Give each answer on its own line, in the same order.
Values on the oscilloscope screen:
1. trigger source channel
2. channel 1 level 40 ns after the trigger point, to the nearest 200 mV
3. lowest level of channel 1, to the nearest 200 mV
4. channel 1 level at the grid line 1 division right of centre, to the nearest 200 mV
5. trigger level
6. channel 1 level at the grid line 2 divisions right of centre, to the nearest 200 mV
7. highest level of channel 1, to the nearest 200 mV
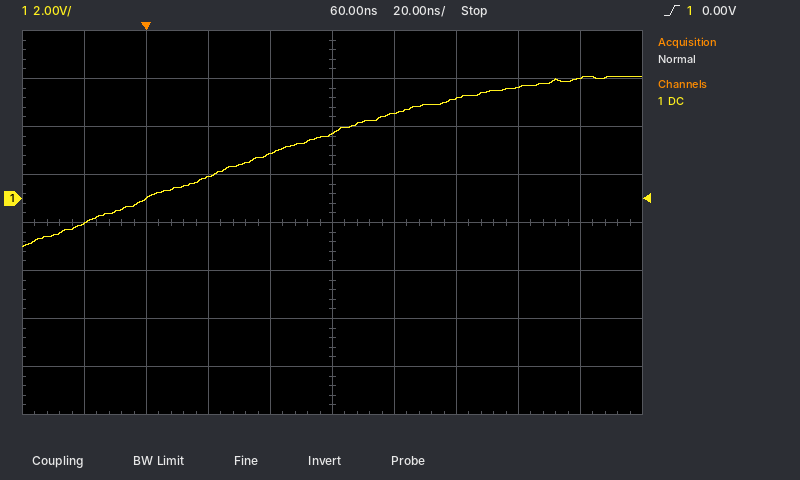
channel 1
1.8 V
-2.0 V
3.6 V
0.00 V
4.2 V
5.0 V
